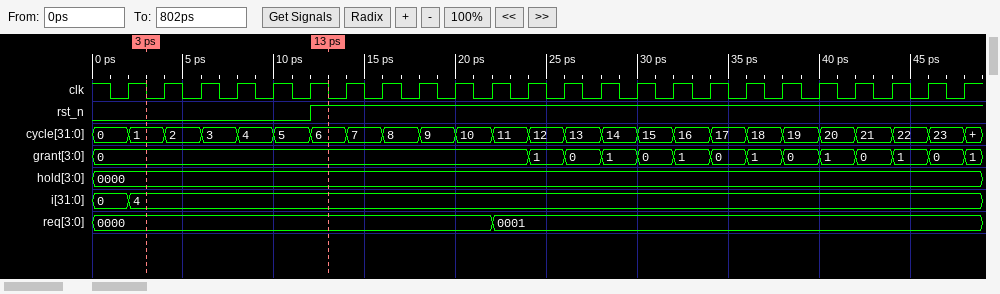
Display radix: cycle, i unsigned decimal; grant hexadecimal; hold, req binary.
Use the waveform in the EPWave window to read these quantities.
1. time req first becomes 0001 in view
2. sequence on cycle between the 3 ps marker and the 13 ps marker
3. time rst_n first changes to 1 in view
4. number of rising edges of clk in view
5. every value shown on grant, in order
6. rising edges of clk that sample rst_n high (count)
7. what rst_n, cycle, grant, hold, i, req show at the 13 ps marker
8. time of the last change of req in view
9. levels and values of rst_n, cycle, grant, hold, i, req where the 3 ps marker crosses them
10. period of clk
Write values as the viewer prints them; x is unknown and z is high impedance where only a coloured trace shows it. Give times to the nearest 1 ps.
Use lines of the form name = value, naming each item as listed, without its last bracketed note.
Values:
time req first becomes 0001 in view = 22 ps
sequence on cycle between the 3 ps marker and the 13 ps marker = 1, 2, 3, 4, 5, 6
time rst_n first changes to 1 in view = 12 ps
number of rising edges of clk in view = 24
every value shown on grant, in order = 0, 1, 0, 1, 0, 1, 0, 1, 0, 1, 0, 1, 0, 1
rising edges of clk that sample rst_n high = 18
what rst_n, cycle, grant, hold, i, req show at the 13 ps marker = rst_n=1, cycle=6, grant=0, hold=0000, i=4, req=0000
time of the last change of req in view = 22 ps
levels and values of rst_n, cycle, grant, hold, i, req where the 3 ps marker crosses them = rst_n=0, cycle=1, grant=0, hold=0000, i=4, req=0000
period of clk = 2 ps
